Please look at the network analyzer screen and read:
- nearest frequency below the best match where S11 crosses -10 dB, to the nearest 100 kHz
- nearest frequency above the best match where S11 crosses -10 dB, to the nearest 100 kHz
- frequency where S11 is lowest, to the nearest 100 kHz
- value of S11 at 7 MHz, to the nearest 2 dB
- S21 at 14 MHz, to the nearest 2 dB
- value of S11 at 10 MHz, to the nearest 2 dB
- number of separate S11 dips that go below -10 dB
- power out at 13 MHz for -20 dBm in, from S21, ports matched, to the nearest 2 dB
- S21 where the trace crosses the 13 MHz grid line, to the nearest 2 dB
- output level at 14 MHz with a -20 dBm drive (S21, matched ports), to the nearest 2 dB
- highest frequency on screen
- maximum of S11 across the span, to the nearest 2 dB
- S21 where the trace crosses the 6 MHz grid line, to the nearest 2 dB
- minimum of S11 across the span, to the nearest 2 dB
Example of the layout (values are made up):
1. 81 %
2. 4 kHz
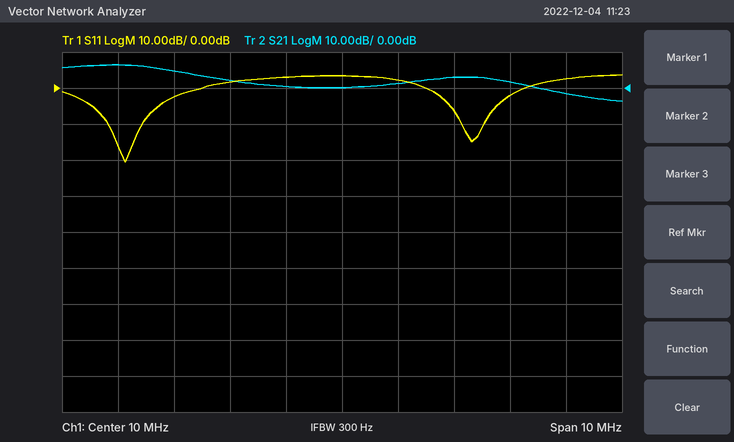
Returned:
1. 5.8 MHz
2. 6.4 MHz
3. 6.1 MHz
4. -2 dB
5. -2 dB
6. 4 dB
7. 2
8. -18 dBm
9. 2 dB
10. -22 dBm
11. 15 MHz
12. 4 dB
13. 6 dB
14. -20 dB
